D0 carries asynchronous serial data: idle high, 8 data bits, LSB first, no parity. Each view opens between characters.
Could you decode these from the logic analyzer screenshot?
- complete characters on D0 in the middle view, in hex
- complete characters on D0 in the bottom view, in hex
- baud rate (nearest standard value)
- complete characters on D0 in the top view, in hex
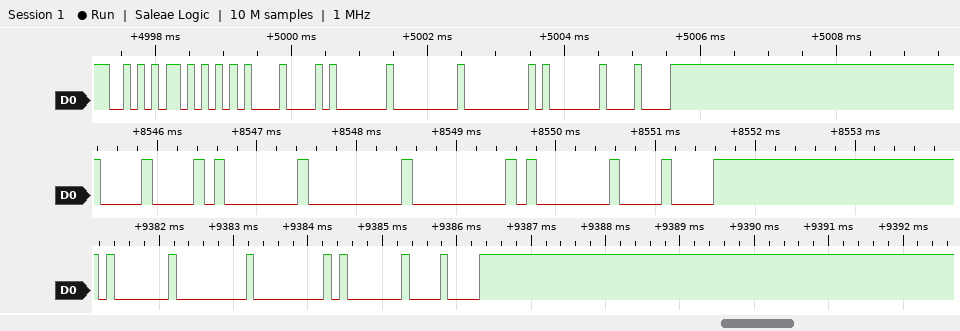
08, 01, 00, 00, 01, 08
01, 00, 00, 01, 08
9600 baud
AA, 55, 08, 01, 00, 00, 01, 08
